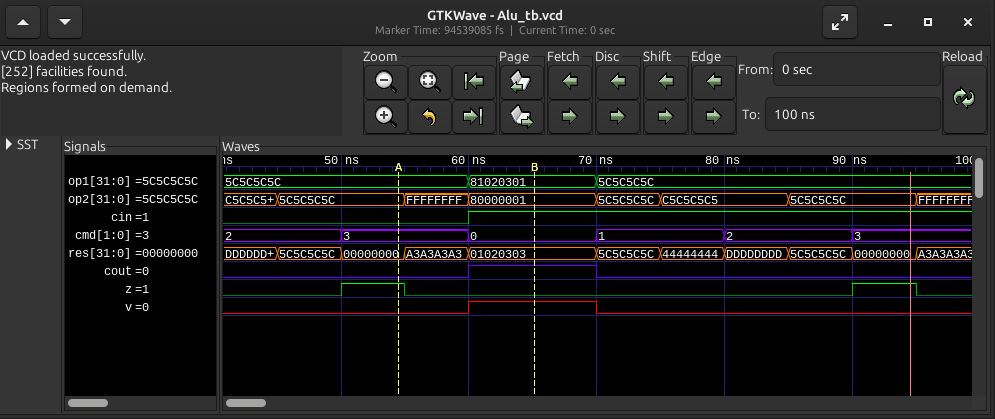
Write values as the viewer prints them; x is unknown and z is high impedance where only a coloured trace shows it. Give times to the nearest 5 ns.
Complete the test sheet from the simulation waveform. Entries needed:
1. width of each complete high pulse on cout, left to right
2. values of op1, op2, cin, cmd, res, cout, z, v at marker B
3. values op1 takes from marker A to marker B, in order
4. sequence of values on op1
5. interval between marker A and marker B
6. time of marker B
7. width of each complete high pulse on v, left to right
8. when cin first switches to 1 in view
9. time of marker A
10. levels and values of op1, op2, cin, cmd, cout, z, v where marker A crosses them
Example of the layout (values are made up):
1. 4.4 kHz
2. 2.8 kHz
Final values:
1. 10 ns
2. op1=81020301, op2=80000001, cin=1, cmd=0, res=01020303, cout=1, z=0, v=1
3. 5C5C5C5C, 81020301
4. 5C5C5C5C, 81020301, 5C5C5C5C
5. 10 ns
6. 65 ns
7. 10 ns
8. 60 ns
9. 55 ns
10. op1=5C5C5C5C, op2=5C5C5C5C, cin=0, cmd=3, cout=0, z=1, v=0
